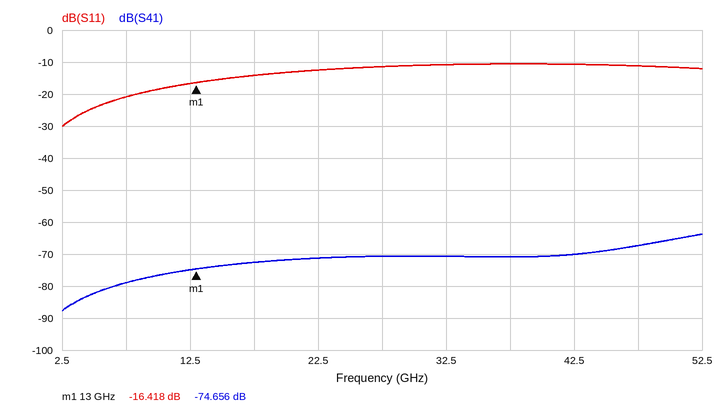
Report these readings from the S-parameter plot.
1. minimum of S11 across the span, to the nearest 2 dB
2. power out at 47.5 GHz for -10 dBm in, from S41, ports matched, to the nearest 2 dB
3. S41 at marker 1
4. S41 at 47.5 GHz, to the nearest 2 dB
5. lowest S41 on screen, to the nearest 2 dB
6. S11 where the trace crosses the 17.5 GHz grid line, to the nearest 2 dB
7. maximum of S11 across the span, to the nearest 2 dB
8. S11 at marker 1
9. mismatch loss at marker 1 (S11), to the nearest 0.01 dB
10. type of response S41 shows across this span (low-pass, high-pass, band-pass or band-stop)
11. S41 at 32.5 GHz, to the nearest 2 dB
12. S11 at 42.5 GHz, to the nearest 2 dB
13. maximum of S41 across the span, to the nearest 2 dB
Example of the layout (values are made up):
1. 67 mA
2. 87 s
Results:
1. -30 dB
2. -78 dBm
3. -74.656 dB
4. -68 dB
5. -88 dB
6. -14 dB
7. -10 dB
8. -16.418 dB
9. 0.10 dB
10. high-pass
11. -70 dB
12. -10 dB
13. -64 dB
